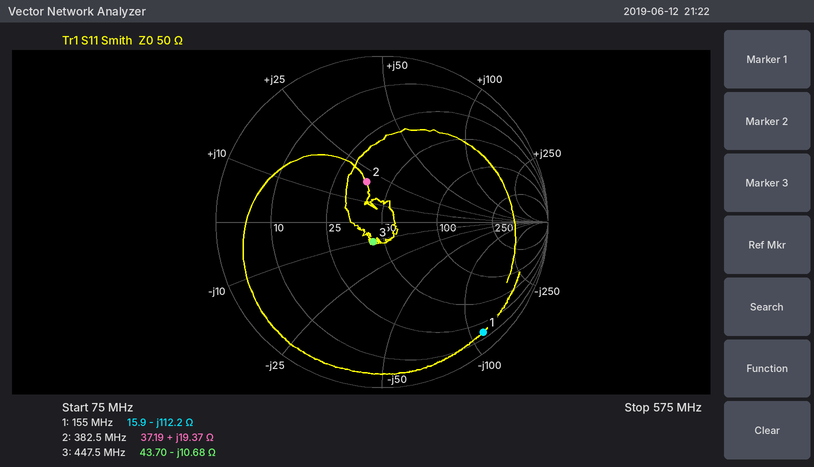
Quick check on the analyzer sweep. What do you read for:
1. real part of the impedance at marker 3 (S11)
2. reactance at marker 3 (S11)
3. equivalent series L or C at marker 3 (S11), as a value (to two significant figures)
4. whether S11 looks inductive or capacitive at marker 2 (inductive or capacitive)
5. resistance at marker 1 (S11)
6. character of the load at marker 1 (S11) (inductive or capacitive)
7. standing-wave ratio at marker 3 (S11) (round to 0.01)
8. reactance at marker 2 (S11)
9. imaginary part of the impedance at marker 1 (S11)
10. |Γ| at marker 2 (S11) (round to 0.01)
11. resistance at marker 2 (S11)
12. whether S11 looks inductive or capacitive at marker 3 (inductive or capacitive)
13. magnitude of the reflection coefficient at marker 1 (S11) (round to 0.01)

43.70 Ω
-10.68 Ω
33 pF
inductive
15.9 Ω
capacitive
1.30
+19.37 Ω
-112.2 Ω
0.26
37.19 Ω
capacitive
0.90
